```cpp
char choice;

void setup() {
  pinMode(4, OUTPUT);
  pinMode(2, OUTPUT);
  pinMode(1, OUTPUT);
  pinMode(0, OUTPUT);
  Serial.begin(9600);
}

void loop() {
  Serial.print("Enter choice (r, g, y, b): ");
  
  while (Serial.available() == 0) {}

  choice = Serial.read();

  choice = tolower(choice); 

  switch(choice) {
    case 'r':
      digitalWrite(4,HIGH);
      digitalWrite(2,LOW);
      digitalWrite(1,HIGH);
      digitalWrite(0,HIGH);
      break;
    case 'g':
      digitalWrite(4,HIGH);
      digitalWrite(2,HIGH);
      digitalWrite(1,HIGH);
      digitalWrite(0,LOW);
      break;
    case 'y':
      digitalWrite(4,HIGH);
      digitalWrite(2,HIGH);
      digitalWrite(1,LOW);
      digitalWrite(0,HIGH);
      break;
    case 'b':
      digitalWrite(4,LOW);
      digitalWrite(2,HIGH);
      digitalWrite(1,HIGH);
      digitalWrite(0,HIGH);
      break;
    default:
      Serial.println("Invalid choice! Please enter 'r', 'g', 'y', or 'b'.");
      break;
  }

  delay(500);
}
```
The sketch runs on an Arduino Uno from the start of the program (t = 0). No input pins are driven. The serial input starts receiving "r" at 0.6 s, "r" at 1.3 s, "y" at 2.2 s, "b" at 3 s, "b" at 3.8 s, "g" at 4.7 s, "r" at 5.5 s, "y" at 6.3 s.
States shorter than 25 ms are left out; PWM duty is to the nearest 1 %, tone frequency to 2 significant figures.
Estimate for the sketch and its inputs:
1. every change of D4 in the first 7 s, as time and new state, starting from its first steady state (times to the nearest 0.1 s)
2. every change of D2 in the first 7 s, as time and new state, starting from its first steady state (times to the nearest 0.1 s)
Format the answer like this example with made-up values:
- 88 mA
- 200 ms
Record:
- 0 s low; 0.6 s high; 3 s low; 4.7 s high
- 0 s low; 2.2 s high; 5.5 s low; 6.3 s high
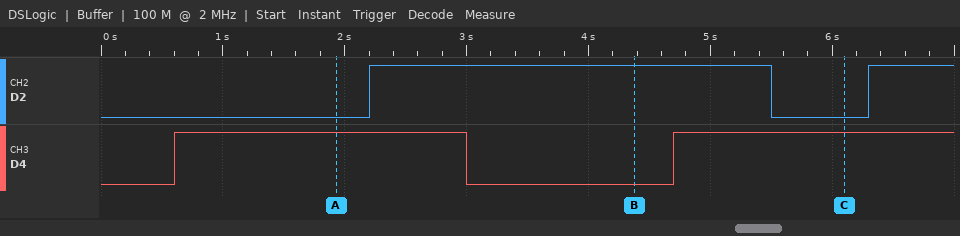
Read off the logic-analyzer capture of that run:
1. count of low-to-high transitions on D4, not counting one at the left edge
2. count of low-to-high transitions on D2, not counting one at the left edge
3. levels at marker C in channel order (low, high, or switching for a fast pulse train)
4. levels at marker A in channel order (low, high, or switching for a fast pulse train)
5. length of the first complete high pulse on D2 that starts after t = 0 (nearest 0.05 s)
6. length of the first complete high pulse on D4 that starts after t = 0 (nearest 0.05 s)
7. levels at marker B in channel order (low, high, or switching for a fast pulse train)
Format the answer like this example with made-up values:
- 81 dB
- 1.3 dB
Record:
- 2
- 2
- D2 low, D4 high
- D2 low, D4 high
- 3.30 s
- 2.40 s
- D2 high, D4 low
